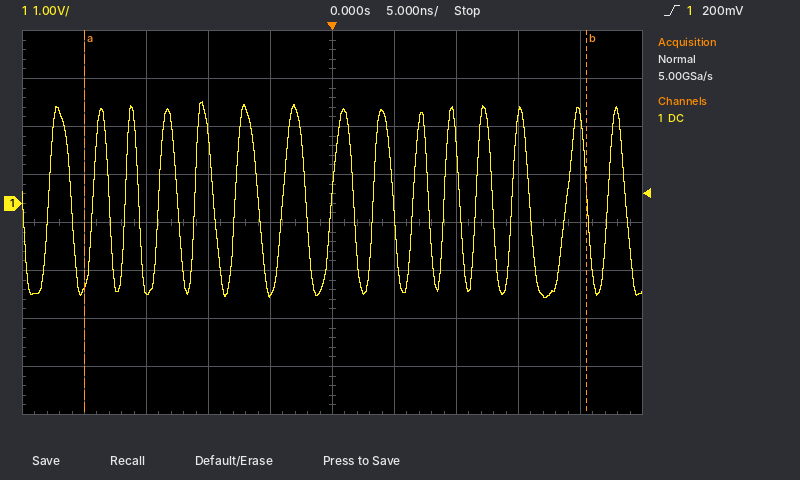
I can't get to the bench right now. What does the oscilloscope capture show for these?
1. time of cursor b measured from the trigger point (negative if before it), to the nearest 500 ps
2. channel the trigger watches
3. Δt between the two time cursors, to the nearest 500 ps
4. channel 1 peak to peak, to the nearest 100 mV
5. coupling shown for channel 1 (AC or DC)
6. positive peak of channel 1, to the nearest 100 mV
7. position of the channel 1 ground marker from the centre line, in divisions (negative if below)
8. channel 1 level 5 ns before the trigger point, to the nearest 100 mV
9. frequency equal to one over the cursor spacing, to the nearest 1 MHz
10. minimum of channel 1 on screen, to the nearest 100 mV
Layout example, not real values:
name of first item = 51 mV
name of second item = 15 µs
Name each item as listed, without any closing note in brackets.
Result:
time of cursor b measured from the trigger point (negative if before it), to the nearest 500 ps = +20.5 ns
channel the trigger watches = channel 1
Δt between the two time cursors, to the nearest 500 ps = 40.5 ns
channel 1 peak to peak, to the nearest 100 mV = 4.1 V
coupling shown for channel 1 = DC
positive peak of channel 1, to the nearest 100 mV = 2.1 V
position of the channel 1 ground marker from the centre line, in divisions = +0.4 div
channel 1 level 5 ns before the trigger point, to the nearest 100 mV = -1.9 V
frequency equal to one over the cursor spacing, to the nearest 1 MHz = 25 MHz
minimum of channel 1 on screen, to the nearest 100 mV = -2.0 V
